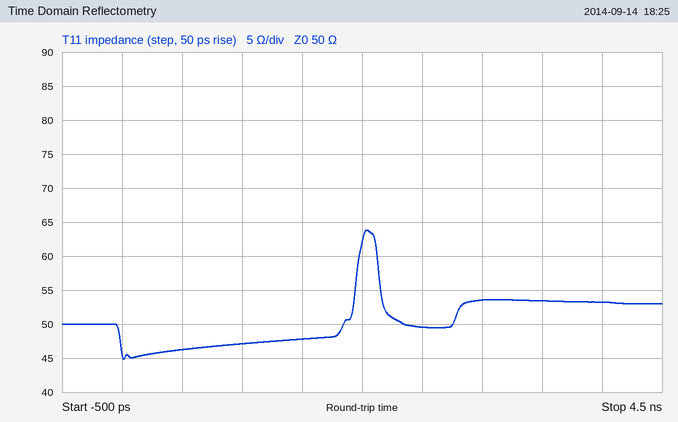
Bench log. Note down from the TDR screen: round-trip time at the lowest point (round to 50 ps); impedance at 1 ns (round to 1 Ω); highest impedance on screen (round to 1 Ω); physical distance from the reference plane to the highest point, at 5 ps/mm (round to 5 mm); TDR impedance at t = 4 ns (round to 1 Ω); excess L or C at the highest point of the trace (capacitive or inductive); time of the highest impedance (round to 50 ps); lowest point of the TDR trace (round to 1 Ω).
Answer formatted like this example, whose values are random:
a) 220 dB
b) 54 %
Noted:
a) 0 ps
b) 47 Ω
c) 64 Ω
d) 205 mm
e) 53 Ω
f) inductive
g) 2.05 ns
h) 45 Ω
